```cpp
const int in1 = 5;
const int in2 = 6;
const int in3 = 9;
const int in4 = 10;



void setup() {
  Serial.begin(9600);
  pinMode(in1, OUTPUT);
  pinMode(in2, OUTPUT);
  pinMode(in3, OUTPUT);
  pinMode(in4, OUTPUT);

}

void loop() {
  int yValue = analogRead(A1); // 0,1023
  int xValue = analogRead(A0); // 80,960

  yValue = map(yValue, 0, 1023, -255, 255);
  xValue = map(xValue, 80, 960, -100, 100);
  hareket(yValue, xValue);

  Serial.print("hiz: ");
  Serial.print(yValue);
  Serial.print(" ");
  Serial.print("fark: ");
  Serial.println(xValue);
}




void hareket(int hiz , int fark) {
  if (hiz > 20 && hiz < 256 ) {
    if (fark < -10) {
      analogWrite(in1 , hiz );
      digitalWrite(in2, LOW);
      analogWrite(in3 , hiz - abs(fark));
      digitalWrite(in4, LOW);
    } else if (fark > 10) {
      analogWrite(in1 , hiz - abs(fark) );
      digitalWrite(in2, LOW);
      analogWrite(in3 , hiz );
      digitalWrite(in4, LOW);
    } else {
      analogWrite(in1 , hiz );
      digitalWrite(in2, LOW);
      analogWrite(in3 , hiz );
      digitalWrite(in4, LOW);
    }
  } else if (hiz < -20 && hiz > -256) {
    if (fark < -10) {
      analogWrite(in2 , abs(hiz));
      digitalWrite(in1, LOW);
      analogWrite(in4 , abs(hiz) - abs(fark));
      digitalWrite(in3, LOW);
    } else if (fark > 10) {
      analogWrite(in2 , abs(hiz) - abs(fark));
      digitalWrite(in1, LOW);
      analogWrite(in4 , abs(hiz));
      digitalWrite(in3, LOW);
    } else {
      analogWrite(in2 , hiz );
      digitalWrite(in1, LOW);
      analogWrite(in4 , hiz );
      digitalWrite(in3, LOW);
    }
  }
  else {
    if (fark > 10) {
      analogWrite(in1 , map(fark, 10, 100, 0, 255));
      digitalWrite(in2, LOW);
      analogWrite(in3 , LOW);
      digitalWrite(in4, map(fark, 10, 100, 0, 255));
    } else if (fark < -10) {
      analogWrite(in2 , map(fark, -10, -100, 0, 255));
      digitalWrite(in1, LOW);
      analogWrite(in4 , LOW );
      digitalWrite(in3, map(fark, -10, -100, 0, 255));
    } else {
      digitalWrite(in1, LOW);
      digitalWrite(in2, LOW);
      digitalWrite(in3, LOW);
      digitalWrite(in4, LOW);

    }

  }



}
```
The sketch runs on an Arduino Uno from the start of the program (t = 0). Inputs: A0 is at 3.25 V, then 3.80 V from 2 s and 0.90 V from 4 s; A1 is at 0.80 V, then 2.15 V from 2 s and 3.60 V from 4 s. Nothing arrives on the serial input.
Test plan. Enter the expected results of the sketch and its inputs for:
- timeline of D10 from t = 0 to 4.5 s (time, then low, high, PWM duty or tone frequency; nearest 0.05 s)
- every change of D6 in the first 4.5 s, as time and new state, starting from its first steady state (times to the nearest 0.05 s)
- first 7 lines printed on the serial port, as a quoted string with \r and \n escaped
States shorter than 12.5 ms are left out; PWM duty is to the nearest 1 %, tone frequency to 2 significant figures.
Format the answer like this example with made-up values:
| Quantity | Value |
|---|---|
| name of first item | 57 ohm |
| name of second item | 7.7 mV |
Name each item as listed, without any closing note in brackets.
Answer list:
| Quantity | Value |
|---|---|
| timeline of D10 from t = 0 to 4.5 s | 0 s PWM 68 %; 2 s PWM 14 %; 4 s low |
| every change of D6 in the first 4.5 s, as time and new state, starting from its first steady state | 0 s PWM 56 %; 2 s PWM 92 %; 4 s low |
| first 7 lines printed on the serial port, as a quoted string with \r and \n escaped | "hiz: -174 fark: 32\r\nhiz: -174 fark: 32\r\nhiz: -174 fark: 32\r\nhiz: -174 fark: 32\r\nhiz: -174 fark: 32\r\nhiz: -174 fark: 32\r\nhiz: -174 fark: 32\r\n" |
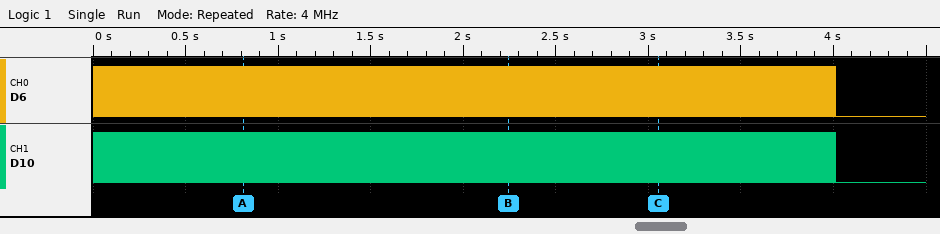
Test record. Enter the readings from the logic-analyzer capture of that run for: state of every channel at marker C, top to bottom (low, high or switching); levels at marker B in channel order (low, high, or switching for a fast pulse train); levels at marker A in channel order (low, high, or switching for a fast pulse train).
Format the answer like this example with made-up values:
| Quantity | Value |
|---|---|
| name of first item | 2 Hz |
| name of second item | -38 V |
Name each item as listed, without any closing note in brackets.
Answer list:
| Quantity | Value |
|---|---|
| state of every channel at marker C, top to bottom | D6 switching, D10 switching |
| levels at marker B in channel order | D6 switching, D10 switching |
| levels at marker A in channel order | D6 switching, D10 switching |
